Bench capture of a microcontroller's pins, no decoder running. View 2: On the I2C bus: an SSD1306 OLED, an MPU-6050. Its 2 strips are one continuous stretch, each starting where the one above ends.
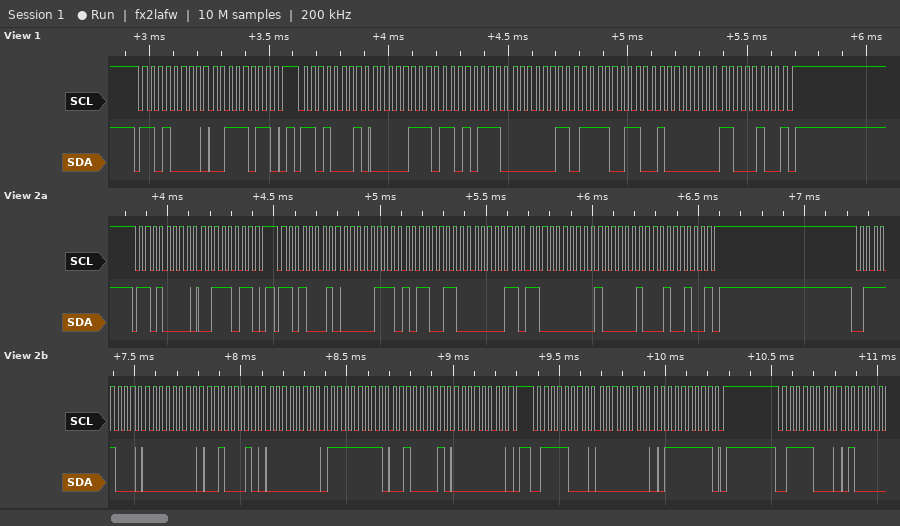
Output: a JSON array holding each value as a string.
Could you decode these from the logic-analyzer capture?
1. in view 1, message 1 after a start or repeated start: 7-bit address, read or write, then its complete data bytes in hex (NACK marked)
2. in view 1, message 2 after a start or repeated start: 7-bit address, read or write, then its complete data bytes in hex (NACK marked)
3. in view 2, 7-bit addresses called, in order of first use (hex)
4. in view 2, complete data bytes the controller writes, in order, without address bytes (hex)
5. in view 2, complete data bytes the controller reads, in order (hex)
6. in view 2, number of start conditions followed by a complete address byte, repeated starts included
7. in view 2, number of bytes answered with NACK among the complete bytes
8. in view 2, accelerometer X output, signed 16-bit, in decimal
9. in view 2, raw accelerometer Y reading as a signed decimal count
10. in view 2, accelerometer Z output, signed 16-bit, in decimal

["0x68 write: 3B", "0x68 read: 07 D7 03 F3 40 C4 NACK", "0x68 0x3C", "3B 00 22 00 FF 21 00 00 7F", "07 B3 03 C0 41 24", "5", "1", "1971", "960", "16676"]
